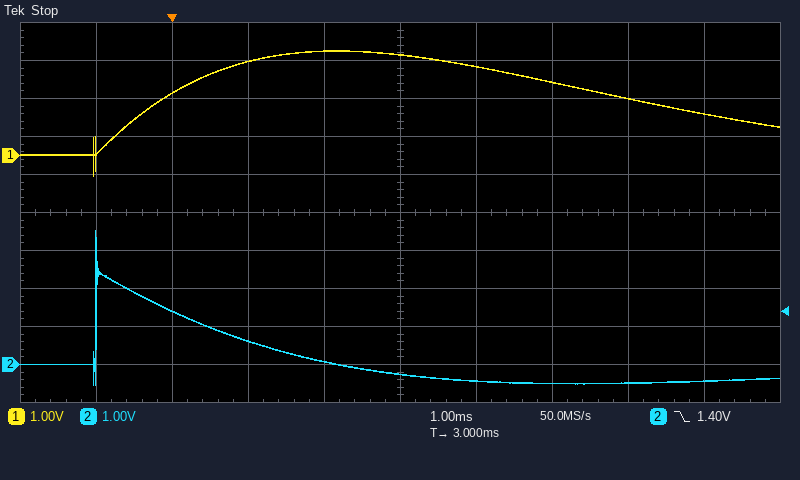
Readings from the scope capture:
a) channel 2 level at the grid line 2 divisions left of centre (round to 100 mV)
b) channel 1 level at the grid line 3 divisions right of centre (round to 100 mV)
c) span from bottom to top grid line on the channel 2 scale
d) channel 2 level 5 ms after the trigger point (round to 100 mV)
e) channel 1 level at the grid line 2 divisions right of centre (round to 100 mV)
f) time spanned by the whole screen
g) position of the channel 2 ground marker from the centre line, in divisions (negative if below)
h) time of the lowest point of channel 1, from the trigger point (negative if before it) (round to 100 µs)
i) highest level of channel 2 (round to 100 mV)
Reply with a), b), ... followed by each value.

a) 600 mV
b) 1.5 V
c) 10 V
d) -500 mV
e) 1.9 V
f) 10 ms
g) -4.0 div
h) -1.0 ms
i) 3.5 V
